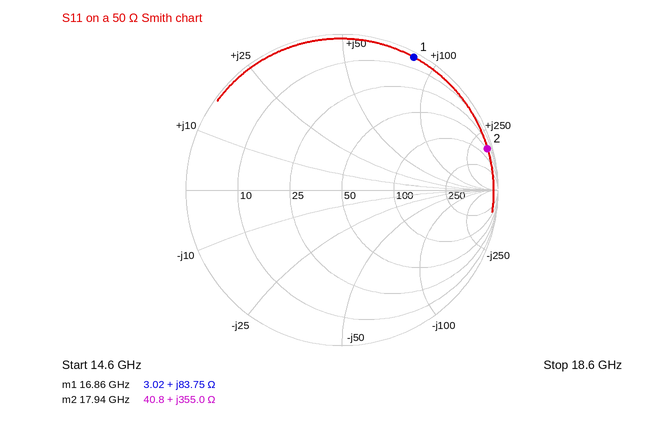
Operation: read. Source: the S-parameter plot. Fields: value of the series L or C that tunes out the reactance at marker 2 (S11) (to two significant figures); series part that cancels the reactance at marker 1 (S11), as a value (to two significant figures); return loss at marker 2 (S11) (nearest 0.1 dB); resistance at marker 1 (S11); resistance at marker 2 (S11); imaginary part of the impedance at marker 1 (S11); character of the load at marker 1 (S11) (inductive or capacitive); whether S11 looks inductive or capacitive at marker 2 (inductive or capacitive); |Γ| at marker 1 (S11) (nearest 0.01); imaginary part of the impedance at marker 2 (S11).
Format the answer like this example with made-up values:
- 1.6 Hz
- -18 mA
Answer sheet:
- 25 fF
- 110 fF
- 0.3 dB
- 3.02 Ω
- 40.8 Ω
- +83.75 Ω
- inductive
- inductive
- 0.97
- +355.0 Ω
